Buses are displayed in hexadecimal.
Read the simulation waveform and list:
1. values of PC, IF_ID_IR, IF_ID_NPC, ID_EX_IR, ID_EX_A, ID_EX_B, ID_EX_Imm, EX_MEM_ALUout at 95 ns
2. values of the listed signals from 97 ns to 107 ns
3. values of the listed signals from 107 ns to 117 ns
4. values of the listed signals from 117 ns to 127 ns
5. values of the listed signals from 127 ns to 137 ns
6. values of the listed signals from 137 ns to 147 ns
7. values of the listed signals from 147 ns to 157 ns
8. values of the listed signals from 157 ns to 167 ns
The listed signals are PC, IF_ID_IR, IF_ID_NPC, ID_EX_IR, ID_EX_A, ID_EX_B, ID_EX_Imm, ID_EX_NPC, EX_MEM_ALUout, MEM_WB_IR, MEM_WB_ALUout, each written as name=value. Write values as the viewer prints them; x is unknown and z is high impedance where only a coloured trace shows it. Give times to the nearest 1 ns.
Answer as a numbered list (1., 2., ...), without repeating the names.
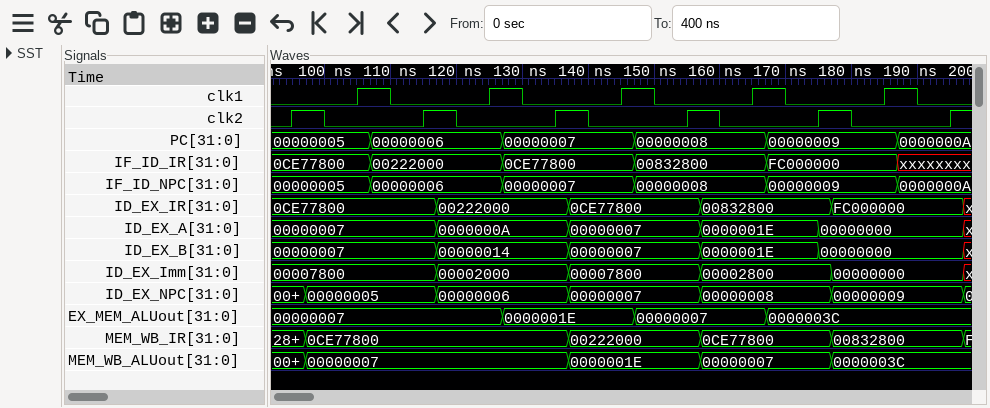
1. PC=00000005, IF_ID_IR=0CE77800, IF_ID_NPC=00000005, ID_EX_IR=0CE77800, ID_EX_A=00000007, ID_EX_B=00000007, ID_EX_Imm=00007800, EX_MEM_ALUout=00000007
2. PC=00000005, IF_ID_IR=0CE77800, IF_ID_NPC=00000005, ID_EX_IR=0CE77800, ID_EX_A=00000007, ID_EX_B=00000007, ID_EX_Imm=00007800, ID_EX_NPC=00000005, EX_MEM_ALUout=00000007, MEM_WB_IR=0CE77800, MEM_WB_ALUout=00000007
3. PC=00000006, IF_ID_IR=00222000, IF_ID_NPC=00000006, ID_EX_IR=0CE77800, ID_EX_A=00000007, ID_EX_B=00000007, ID_EX_Imm=00007800, ID_EX_NPC=00000005, EX_MEM_ALUout=00000007, MEM_WB_IR=0CE77800, MEM_WB_ALUout=00000007
4. PC=00000006, IF_ID_IR=00222000, IF_ID_NPC=00000006, ID_EX_IR=00222000, ID_EX_A=0000000A, ID_EX_B=00000014, ID_EX_Imm=00002000, ID_EX_NPC=00000006, EX_MEM_ALUout=00000007, MEM_WB_IR=0CE77800, MEM_WB_ALUout=00000007
5. PC=00000007, IF_ID_IR=0CE77800, IF_ID_NPC=00000007, ID_EX_IR=00222000, ID_EX_A=0000000A, ID_EX_B=00000014, ID_EX_Imm=00002000, ID_EX_NPC=00000006, EX_MEM_ALUout=0000001E, MEM_WB_IR=0CE77800, MEM_WB_ALUout=00000007
6. PC=00000007, IF_ID_IR=0CE77800, IF_ID_NPC=00000007, ID_EX_IR=0CE77800, ID_EX_A=00000007, ID_EX_B=00000007, ID_EX_Imm=00007800, ID_EX_NPC=00000007, EX_MEM_ALUout=0000001E, MEM_WB_IR=00222000, MEM_WB_ALUout=0000001E
7. PC=00000008, IF_ID_IR=00832800, IF_ID_NPC=00000008, ID_EX_IR=0CE77800, ID_EX_A=00000007, ID_EX_B=00000007, ID_EX_Imm=00007800, ID_EX_NPC=00000007, EX_MEM_ALUout=00000007, MEM_WB_IR=00222000, MEM_WB_ALUout=0000001E
8. PC=00000008, IF_ID_IR=00832800, IF_ID_NPC=00000008, ID_EX_IR=00832800, ID_EX_A=0000001E, ID_EX_B=0000001E, ID_EX_Imm=00002800, ID_EX_NPC=00000008, EX_MEM_ALUout=00000007, MEM_WB_IR=0CE77800, MEM_WB_ALUout=00000007
